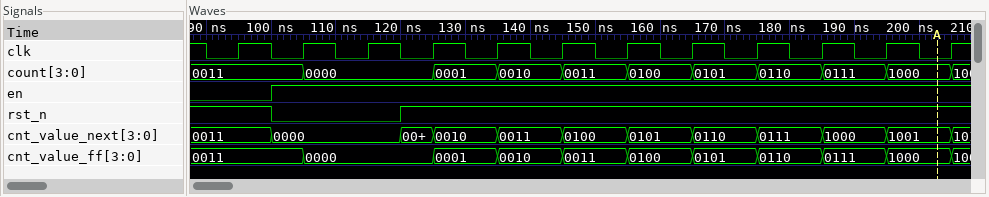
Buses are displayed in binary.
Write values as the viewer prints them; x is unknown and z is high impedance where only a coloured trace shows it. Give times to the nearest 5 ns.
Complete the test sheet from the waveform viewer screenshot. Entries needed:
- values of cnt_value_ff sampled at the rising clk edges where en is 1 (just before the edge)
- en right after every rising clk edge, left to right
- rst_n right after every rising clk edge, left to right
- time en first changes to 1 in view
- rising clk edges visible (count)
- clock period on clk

0011, 0000, 0000, 0001, 0010, 0011, 0100, 0101, 0110, 0111, 1000
0 1 1 1 1 1 1 1 1 1 1 1
1 0 0 1 1 1 1 1 1 1 1 1
100 ns
12
10 ns
